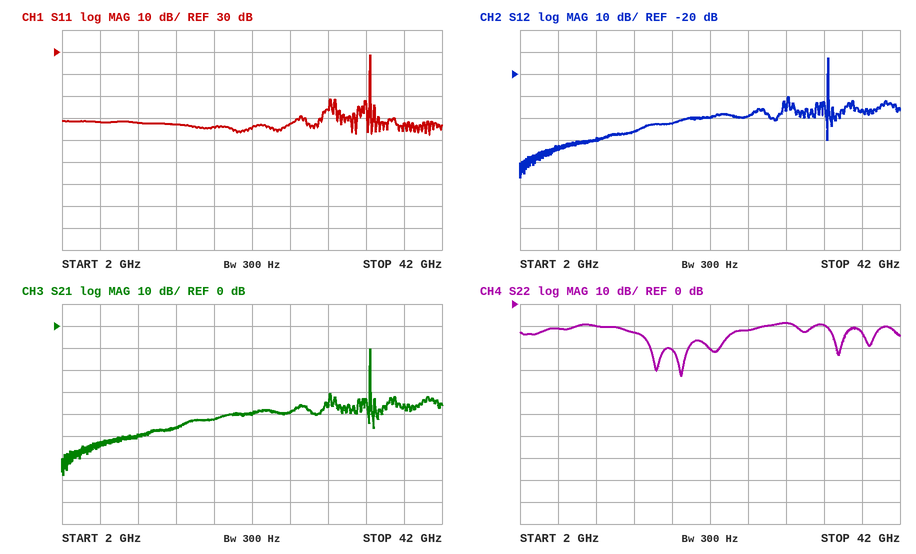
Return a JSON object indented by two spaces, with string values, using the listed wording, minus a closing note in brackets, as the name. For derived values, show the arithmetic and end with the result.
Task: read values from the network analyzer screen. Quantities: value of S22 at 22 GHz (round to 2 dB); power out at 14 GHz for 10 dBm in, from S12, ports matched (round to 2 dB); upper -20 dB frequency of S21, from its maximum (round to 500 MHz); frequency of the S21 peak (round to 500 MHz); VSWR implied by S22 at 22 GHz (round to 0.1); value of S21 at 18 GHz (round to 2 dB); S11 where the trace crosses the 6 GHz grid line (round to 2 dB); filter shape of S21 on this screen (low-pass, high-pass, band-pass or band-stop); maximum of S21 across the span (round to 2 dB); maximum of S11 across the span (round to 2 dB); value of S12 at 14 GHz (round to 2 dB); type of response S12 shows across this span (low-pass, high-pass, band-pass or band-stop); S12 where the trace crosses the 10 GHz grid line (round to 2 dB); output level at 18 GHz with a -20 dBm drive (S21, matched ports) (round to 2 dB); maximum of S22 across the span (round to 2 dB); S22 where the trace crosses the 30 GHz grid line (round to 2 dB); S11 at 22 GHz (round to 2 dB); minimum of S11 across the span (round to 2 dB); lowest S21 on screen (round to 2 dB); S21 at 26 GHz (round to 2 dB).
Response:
{
  "value of S22 at 22 GHz": "-20 dB",
  "power out at 14 GHz for 10 dBm in, from S12, ports matched": "10 dBm + (-46 dB) = -36 dBm",
  "upper -20 dB frequency of S21, from its maximum": "34.5 GHz",
  "frequency of the S21 peak": "34.5 GHz",
  "VSWR implied by S22 at 22 GHz": "|Γ| = 10^(-20/20) = 0.1000; VSWR = (1 + 0.1000)/(1 − 0.1000) ≈ 1.2",
  "value of S21 at 18 GHz": "-42 dB",
  "S11 where the trace crosses the 6 GHz grid line": "-2 dB",
  "filter shape of S21 on this screen": "band-pass",
  "maximum of S21 across the span": "-10 dB",
  "maximum of S11 across the span": "28 dB",
  "value of S12 at 14 GHz": "-46 dB",
  "type of response S12 shows across this span": "band-pass",
  "S12 where the trace crosses the 10 GHz grid line": "-50 dB",
  "output level at 18 GHz with a -20 dBm drive (S21, matched ports)": "-20 dBm + (-42 dB) = -62 dBm",
  "maximum of S22 across the span": "-8 dB",
  "S22 where the trace crosses the 30 GHz grid line": "-8 dB",
  "S11 at 22 GHz": "-4 dB",
  "minimum of S11 across the span": "-8 dB",
  "lowest S21 on screen": "-68 dB",
  "S21 at 26 GHz": "-40 dB"
}
